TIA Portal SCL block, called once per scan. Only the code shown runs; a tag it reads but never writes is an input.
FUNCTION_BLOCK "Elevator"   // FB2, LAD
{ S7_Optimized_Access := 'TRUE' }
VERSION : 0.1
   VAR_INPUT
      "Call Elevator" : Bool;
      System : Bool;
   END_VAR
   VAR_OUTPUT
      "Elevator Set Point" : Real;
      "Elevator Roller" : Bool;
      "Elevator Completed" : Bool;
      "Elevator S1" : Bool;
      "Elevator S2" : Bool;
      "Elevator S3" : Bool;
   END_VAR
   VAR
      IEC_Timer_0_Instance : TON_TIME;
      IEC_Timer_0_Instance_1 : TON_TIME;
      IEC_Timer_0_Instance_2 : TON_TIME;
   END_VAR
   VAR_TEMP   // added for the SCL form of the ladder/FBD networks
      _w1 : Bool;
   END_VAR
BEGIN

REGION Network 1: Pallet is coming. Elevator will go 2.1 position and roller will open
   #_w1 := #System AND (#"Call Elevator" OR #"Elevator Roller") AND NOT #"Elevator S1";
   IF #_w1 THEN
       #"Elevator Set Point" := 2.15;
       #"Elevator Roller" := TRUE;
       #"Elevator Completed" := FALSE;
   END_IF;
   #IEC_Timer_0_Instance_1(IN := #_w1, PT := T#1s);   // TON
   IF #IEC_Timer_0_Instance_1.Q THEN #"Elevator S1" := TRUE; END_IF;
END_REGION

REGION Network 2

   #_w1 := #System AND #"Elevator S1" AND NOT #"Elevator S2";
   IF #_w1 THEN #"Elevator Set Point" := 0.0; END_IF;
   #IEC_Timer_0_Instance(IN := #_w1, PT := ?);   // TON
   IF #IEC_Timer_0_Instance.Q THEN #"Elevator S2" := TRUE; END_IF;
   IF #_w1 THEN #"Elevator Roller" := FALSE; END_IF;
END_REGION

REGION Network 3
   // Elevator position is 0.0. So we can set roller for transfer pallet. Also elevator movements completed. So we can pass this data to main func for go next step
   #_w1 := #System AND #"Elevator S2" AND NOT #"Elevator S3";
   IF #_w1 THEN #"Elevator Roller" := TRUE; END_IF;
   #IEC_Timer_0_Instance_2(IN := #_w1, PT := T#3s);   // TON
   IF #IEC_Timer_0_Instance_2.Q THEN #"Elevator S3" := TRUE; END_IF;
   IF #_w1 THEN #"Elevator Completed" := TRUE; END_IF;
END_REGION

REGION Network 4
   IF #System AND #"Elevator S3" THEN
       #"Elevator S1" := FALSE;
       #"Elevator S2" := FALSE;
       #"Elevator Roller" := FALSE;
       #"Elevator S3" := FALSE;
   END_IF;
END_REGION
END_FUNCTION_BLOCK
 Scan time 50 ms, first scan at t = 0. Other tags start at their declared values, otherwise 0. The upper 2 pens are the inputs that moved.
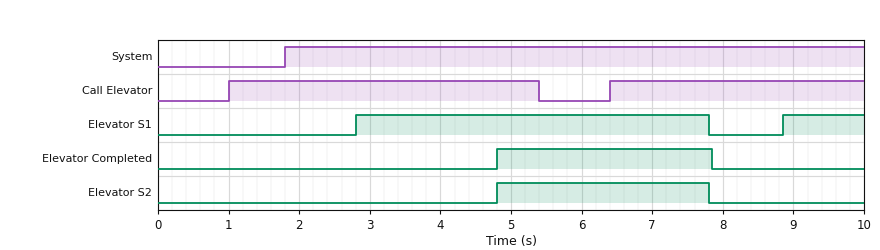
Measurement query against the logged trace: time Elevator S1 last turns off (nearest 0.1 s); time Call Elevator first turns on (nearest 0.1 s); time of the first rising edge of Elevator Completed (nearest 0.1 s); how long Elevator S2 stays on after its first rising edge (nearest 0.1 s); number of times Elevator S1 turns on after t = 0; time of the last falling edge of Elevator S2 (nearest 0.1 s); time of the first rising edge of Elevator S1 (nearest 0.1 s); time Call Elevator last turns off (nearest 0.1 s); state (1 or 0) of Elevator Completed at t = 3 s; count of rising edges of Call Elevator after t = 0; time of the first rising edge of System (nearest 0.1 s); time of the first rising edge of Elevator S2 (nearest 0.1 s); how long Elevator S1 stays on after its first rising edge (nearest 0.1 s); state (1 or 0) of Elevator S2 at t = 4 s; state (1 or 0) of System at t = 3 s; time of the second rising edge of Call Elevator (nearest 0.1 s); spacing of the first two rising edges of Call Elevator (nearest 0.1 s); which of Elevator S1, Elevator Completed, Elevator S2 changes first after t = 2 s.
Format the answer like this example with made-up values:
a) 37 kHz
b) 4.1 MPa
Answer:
a) 7.8 s
b) 1.0 s
c) 4.8 s
d) 3.0 s
e) 2
f) 7.8 s
g) 2.8 s
h) 5.4 s
i) 0
j) 2
k) 1.8 s
l) 4.8 s
m) 5.0 s
n) 0
o) 1
p) 6.4 s
q) 5.4 s
r) Elevator S1
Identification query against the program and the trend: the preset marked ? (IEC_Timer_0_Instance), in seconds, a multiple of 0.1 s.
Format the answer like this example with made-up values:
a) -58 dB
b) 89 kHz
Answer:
a) 2.0 s
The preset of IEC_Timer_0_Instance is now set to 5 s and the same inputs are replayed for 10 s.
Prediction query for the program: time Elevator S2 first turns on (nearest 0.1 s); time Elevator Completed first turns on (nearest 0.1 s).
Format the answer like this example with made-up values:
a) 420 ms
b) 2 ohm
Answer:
a) 7.8 s
b) 7.8 s
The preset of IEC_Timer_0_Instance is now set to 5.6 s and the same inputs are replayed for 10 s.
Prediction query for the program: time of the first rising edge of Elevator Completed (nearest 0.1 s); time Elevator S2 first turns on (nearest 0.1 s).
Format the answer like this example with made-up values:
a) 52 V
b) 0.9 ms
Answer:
a) 8.4 s
b) 8.4 s
